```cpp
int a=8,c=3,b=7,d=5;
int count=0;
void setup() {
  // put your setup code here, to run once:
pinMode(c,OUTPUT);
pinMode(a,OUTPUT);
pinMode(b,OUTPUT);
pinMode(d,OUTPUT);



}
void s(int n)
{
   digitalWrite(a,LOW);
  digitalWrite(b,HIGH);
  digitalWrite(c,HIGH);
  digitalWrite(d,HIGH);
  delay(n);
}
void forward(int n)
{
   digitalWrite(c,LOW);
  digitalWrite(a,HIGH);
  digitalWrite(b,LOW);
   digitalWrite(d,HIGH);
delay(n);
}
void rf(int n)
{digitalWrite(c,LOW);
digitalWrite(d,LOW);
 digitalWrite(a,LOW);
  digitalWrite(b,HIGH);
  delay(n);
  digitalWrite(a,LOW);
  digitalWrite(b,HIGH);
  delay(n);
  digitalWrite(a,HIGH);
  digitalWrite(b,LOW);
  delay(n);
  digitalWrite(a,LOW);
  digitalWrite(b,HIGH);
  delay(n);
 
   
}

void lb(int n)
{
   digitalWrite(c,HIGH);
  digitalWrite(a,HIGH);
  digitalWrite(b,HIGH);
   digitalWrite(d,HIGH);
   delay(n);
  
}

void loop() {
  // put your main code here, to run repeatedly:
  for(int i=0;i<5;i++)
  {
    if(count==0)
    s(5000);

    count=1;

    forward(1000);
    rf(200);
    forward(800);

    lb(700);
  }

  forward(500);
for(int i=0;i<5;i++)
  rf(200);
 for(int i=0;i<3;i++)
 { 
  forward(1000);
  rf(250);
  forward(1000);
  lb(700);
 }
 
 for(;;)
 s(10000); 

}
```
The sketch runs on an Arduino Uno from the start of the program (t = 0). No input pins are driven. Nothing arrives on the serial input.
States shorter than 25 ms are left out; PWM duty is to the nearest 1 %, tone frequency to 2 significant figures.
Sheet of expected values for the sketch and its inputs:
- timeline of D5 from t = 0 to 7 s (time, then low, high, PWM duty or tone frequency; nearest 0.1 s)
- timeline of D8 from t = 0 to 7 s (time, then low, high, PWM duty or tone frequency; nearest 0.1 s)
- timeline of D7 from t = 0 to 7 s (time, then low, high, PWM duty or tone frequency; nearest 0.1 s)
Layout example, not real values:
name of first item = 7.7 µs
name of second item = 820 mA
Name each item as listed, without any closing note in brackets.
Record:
timeline of D5 from t = 0 to 7 s = 0 s high; 6 s low; 6.8 s high
timeline of D8 from t = 0 to 7 s = 0 s low; 5 s high; 6 s low; 6.4 s high; 6.6 s low; 6.8 s high
timeline of D7 from t = 0 to 7 s = 0 s high; 5 s low; 6 s high; 6.4 s low; 6.6 s high; 6.8 s low
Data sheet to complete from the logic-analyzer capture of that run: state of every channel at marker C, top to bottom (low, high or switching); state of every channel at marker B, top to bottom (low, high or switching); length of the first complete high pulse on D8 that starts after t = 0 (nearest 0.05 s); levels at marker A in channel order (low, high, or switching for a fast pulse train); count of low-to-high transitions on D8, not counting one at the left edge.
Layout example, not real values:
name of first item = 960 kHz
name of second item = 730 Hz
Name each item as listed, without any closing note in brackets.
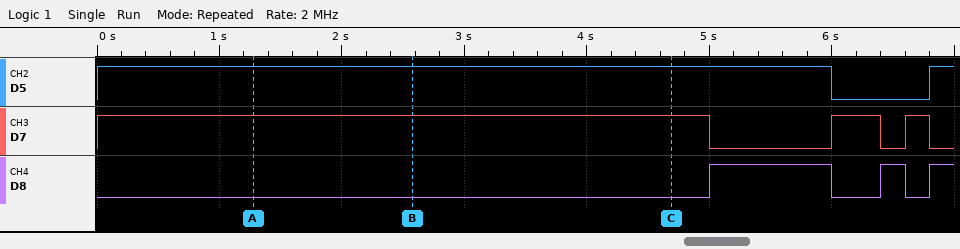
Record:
state of every channel at marker C, top to bottom = D5 high, D7 high, D8 low
state of every channel at marker B, top to bottom = D5 high, D7 high, D8 low
length of the first complete high pulse on D8 that starts after t = 0 = 1.00 s
levels at marker A in channel order = D5 high, D7 high, D8 low
count of low-to-high transitions on D8, not counting one at the left edge = 3
